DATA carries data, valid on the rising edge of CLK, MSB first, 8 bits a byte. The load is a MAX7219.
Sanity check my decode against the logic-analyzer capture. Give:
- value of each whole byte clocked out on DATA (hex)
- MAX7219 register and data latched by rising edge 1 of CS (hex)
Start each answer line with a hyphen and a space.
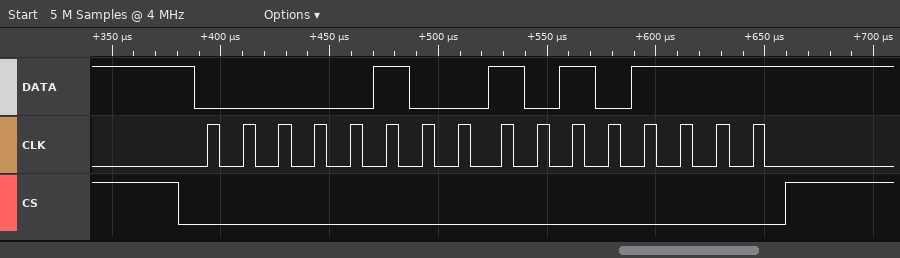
- 04 AF
- register 0x4, data 0xAF
